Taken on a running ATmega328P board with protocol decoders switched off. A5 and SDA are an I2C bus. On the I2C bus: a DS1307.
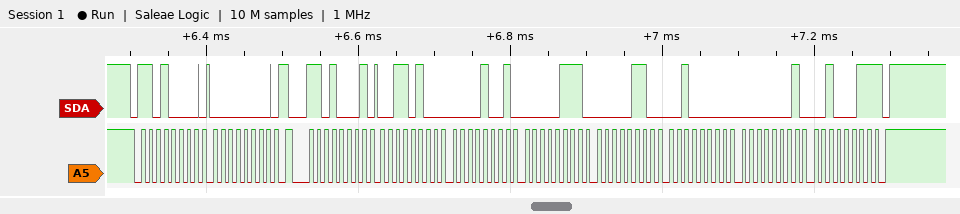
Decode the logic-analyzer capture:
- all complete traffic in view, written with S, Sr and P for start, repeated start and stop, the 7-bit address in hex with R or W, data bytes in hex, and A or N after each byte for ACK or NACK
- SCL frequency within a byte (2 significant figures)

S 68W A 00 A Sr 68R A 34 A 09 A 07 A 06 A 20 A 01 A 23 N P
100 kHz
